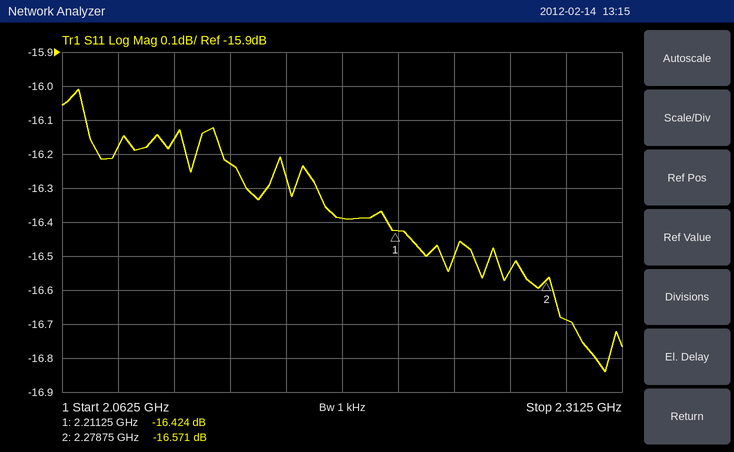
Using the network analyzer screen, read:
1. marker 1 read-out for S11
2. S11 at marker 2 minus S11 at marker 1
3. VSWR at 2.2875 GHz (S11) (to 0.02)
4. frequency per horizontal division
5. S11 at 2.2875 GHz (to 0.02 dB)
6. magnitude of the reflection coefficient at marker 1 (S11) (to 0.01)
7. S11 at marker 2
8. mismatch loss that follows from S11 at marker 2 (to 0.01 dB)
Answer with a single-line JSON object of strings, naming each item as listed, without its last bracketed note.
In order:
{"marker 1 read-out for S11": "-16.424 dB", "S11 at marker 2 minus S11 at marker 1": "-0.147 dB", "VSWR at 2.2875 GHz (S11)": "1.34", "frequency per horizontal division": "25 MHz", "S11 at 2.2875 GHz": "-16.68 dB", "magnitude of the reflection coefficient at marker 1 (S11)": "0.15", "S11 at marker 2": "-16.571 dB", "mismatch loss that follows from S11 at marker 2": "0.10 dB"}
